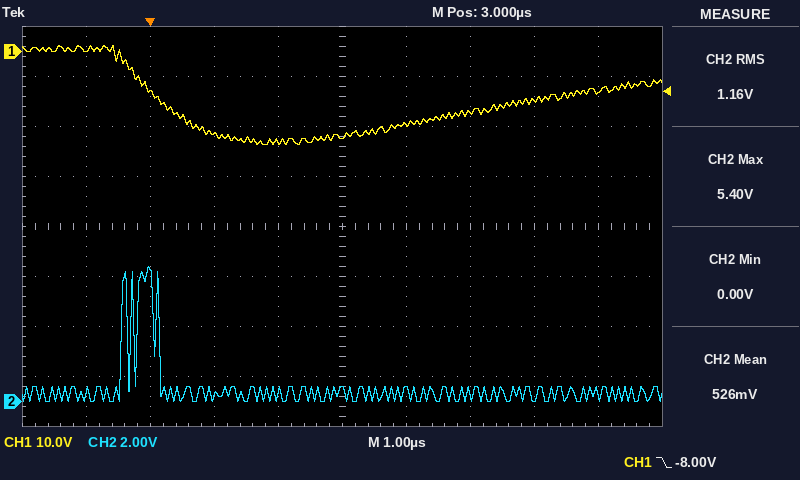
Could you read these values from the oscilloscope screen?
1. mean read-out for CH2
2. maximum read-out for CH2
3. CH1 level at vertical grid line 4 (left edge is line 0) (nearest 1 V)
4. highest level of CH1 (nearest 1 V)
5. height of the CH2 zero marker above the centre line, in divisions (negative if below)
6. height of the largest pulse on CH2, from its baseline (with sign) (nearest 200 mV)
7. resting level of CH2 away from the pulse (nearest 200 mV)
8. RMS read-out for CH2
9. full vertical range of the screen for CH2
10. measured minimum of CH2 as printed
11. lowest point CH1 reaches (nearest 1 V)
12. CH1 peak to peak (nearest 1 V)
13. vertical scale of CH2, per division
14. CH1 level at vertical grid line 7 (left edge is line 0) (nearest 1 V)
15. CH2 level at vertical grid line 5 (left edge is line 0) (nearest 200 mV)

526 mV
5.40 V
-18 V
1 V
-3.5 div
+5.0 V
400 mV
1.16 V
16 V
0.00 V
-19 V
20 V
2 V
-12 V
400 mV
